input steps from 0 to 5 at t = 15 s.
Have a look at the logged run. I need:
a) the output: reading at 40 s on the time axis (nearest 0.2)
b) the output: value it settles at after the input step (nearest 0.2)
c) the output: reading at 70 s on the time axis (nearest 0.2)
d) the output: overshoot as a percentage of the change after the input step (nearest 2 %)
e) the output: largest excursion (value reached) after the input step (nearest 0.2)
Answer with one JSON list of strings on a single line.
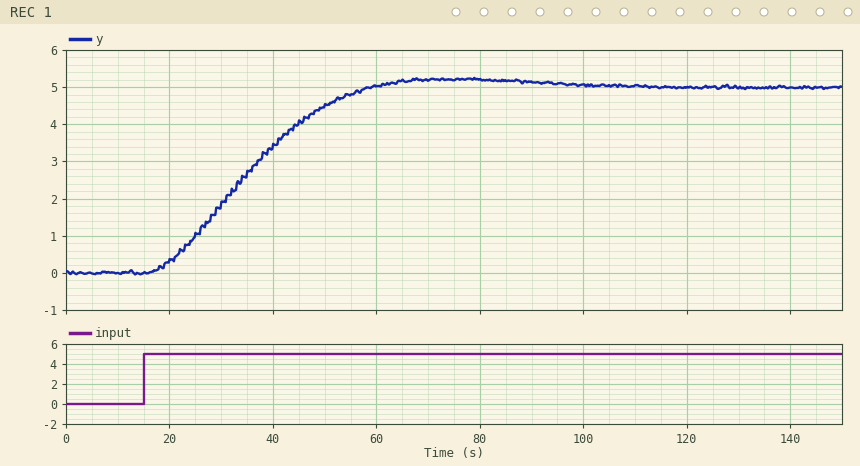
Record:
["3.4", "5.0", "5.2", "4 %", "5.2"]
